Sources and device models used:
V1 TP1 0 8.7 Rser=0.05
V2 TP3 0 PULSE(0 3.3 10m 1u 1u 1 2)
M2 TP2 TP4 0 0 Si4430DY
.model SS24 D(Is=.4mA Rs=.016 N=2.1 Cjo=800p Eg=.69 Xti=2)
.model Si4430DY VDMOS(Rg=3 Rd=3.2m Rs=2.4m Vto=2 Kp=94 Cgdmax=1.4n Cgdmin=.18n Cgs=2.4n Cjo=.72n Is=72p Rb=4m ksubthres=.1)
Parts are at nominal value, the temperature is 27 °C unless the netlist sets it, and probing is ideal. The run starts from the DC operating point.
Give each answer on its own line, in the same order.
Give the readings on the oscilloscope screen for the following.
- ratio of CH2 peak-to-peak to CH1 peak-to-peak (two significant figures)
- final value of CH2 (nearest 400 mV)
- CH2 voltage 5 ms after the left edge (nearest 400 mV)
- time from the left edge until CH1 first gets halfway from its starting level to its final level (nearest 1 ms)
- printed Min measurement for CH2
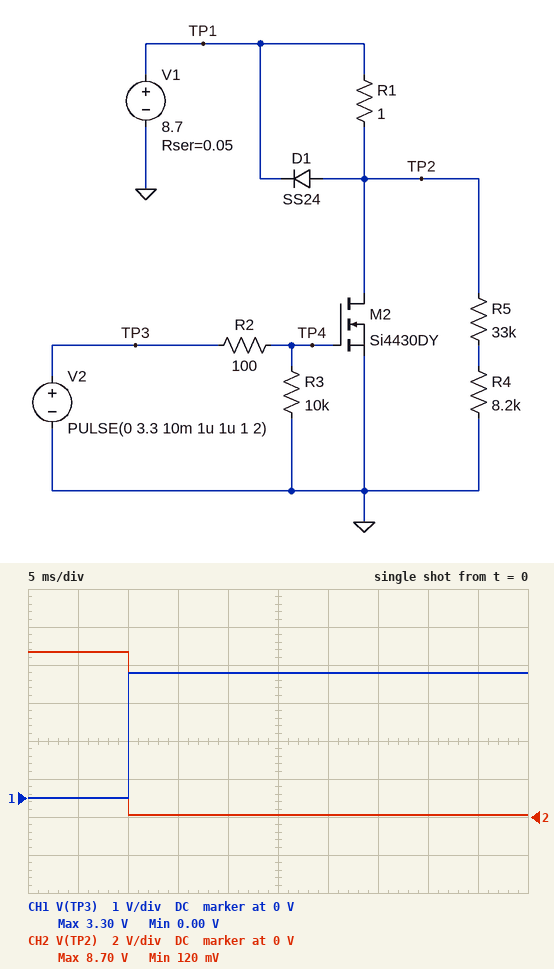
2.6
0 V
8.8 V
10 ms
120 mV
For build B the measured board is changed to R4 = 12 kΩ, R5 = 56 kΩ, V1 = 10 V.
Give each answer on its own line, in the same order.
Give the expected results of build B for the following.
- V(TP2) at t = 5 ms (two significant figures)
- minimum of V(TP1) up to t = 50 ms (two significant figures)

10 V
9.5 V
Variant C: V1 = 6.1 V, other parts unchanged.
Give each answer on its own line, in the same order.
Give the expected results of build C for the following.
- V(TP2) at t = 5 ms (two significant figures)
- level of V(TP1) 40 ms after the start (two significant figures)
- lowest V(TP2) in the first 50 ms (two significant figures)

6.1 V
5.8 V
82 mV
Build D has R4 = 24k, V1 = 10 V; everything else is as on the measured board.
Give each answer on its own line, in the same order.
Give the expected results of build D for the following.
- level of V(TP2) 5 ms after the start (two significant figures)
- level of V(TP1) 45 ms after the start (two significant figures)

10 V
9.5 V
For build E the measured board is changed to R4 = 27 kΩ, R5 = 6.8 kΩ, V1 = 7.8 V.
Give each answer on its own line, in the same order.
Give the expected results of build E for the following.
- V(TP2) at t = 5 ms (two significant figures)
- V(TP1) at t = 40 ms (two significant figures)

7.8 V
7.4 V
